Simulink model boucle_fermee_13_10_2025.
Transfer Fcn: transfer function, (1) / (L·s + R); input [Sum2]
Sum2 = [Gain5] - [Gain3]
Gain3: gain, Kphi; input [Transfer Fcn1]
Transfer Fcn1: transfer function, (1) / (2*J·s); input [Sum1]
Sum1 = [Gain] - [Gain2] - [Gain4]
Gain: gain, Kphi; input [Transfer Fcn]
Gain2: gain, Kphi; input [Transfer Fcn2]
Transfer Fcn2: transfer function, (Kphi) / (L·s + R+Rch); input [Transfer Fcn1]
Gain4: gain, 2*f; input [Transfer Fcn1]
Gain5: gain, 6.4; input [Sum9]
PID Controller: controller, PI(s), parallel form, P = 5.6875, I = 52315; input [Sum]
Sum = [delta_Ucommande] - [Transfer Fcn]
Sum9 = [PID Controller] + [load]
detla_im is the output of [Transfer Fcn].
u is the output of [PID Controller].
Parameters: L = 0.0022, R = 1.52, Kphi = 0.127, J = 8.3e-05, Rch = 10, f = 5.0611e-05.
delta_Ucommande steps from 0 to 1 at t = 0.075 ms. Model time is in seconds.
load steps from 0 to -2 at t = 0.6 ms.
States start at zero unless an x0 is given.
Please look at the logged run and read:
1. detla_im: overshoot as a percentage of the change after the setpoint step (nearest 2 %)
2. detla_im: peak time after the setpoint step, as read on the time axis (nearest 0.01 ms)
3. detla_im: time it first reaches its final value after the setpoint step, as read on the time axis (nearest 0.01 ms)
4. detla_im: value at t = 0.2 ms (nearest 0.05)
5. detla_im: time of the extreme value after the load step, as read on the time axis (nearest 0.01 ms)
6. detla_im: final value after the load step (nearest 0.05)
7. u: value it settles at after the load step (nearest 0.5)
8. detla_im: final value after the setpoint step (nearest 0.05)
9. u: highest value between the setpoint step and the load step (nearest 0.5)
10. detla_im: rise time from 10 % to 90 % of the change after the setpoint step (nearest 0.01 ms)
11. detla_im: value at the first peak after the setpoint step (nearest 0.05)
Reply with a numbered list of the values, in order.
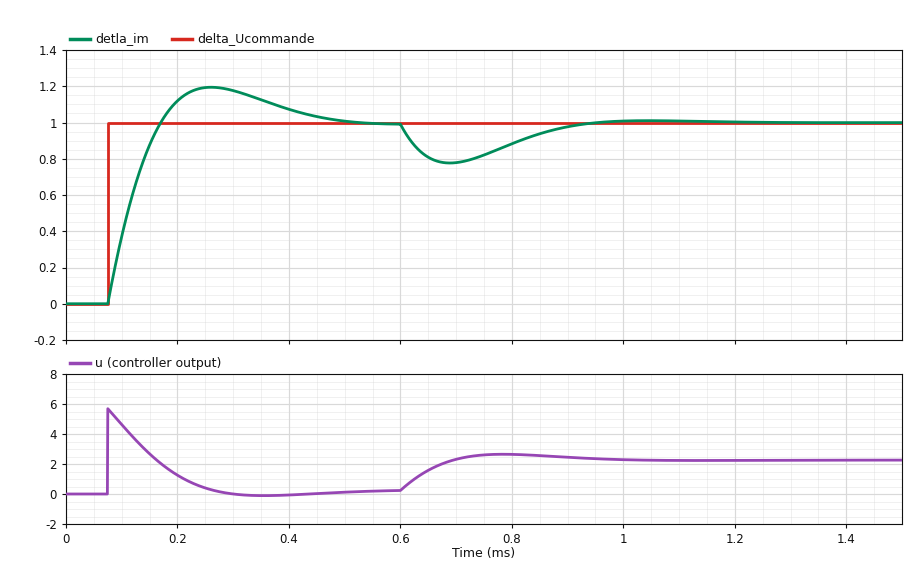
1. 20 %
2. 0.26 ms
3. 0.17 ms
4. 1.10
5. 0.69 ms
6. 1.00
7. 2.5
8. 1.00
9. 5.5
10. 0.07 ms
11. 1.20
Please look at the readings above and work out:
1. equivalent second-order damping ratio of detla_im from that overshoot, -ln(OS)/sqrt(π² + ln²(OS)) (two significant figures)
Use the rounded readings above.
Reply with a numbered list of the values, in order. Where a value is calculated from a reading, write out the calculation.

1. ln(0.2) = -1.609; 1.609 / sqrt(9.870 + 2.590) = 0.46
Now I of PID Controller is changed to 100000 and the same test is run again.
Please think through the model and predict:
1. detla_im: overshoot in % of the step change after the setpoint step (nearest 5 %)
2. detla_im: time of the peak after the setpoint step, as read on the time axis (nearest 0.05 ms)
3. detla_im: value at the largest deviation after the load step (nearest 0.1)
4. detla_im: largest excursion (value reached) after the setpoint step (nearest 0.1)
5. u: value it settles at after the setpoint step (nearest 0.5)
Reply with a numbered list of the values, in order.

1. 30 %
2. 0.20 ms
3. 0.8
4. 1.3
5. 0.5
